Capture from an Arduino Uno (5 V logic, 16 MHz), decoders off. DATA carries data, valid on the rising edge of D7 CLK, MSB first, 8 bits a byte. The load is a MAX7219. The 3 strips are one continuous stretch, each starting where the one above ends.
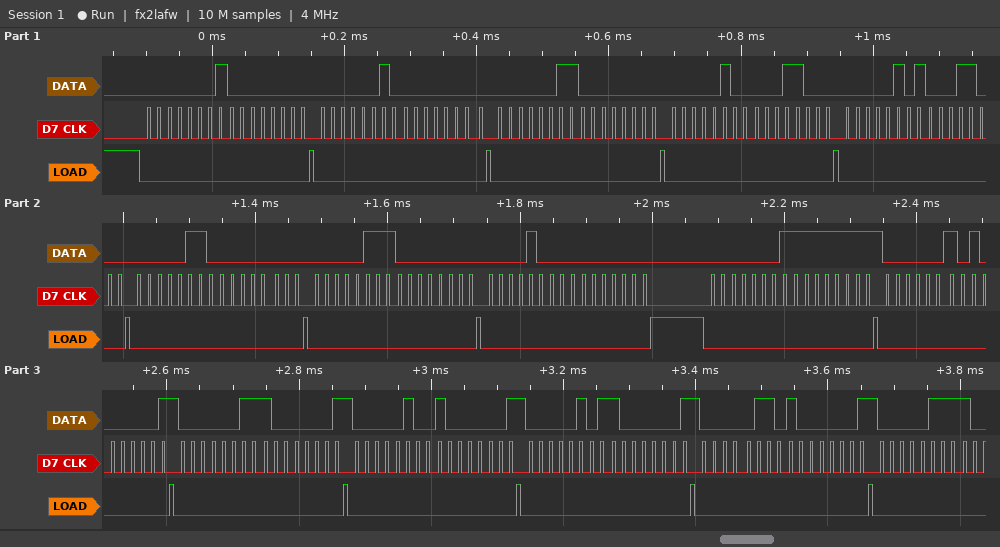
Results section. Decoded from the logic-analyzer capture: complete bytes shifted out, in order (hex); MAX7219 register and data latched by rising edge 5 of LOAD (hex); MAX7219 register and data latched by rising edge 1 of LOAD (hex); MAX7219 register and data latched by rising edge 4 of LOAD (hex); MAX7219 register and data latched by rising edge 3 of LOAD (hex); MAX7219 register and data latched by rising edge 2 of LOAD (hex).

01 00 02 00 03 00 04 18 05 18 06 00 07 00 08 00 01 FF 02 81 03 81 04 81 05 81 06 81 07
register 0x5, data 0x18
register 0x1, data 0x00
register 0x4, data 0x18
register 0x3, data 0x00
register 0x2, data 0x00
